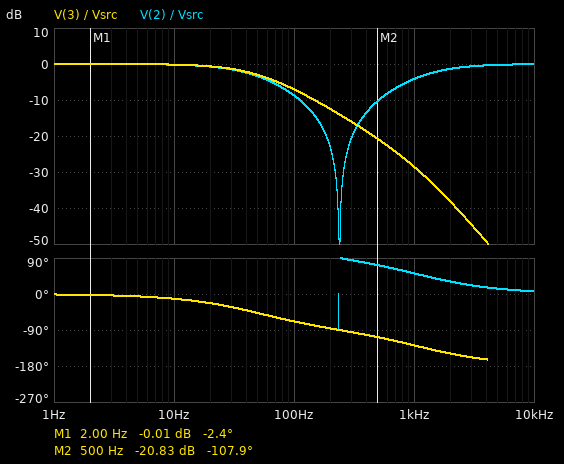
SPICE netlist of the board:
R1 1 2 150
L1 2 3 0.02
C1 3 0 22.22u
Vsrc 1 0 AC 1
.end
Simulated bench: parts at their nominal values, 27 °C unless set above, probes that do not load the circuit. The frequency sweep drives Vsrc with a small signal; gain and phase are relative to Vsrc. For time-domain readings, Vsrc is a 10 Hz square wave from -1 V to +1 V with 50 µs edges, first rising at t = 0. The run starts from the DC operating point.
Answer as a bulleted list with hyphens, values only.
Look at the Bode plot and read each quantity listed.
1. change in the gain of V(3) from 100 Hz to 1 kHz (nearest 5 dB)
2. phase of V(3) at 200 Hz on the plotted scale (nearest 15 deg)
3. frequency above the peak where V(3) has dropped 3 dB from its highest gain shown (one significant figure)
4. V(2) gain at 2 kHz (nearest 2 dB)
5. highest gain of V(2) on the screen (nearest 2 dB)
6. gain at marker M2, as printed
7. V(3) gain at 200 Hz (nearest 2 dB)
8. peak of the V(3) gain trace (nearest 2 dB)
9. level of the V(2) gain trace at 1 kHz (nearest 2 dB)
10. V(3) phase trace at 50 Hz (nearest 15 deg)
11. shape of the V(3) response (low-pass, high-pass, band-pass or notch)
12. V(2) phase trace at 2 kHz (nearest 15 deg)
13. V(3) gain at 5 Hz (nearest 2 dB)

- -20 dB
- -90 deg
- 50 Hz
- -2 dB
- 0 dB
- -20.83 dB
- -12 dB
- 0 dB
- -4 dB
- -45 deg
- low-pass
- 30 deg
- 0 dB
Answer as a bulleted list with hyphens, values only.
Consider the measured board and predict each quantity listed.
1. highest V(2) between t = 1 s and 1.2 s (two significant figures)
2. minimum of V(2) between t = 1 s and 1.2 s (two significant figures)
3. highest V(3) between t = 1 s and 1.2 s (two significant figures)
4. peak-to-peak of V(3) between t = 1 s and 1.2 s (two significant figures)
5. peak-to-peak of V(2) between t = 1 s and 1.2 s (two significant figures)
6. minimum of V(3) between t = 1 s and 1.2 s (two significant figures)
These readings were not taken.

- 1.0 V
- -1.0 V
- 1.0 V
- 2.0 V
- 2.0 V
- -1.0 V
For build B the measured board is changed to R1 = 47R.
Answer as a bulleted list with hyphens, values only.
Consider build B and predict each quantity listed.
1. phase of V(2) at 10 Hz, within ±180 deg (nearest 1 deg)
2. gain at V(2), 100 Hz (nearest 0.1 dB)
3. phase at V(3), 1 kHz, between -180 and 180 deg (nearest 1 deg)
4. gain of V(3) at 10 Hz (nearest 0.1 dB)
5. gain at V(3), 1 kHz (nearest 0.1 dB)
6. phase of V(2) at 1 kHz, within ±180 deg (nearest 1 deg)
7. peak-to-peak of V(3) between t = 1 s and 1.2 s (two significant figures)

- -4 deg
- -2.1 dB
- -158 deg
- 0 dB
- -25.0 dB
- 22 deg
- 2.1 V
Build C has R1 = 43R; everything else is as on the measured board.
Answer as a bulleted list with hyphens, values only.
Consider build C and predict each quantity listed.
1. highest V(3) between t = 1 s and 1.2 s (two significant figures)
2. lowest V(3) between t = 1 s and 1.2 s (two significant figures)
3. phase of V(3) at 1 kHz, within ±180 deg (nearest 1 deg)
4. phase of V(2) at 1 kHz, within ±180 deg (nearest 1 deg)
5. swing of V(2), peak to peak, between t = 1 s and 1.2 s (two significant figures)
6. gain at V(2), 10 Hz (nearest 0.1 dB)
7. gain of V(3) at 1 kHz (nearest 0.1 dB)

- 1.1 V
- -1.1 V
- -160 deg
- 20 deg
- 2.1 V
- 0 dB
- -24.9 dB
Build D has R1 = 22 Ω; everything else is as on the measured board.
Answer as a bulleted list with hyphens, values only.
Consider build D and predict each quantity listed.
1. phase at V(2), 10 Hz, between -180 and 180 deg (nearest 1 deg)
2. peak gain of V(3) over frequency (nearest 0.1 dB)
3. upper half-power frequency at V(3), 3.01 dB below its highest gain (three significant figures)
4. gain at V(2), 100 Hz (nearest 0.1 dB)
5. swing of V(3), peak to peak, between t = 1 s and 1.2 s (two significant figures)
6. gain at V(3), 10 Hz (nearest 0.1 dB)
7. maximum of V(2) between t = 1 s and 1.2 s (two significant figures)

- -2 deg
- 3.3 dB
- 284 Hz
- -0.6 dB
- 3.2 V
- 0 dB
- 1.3 V
